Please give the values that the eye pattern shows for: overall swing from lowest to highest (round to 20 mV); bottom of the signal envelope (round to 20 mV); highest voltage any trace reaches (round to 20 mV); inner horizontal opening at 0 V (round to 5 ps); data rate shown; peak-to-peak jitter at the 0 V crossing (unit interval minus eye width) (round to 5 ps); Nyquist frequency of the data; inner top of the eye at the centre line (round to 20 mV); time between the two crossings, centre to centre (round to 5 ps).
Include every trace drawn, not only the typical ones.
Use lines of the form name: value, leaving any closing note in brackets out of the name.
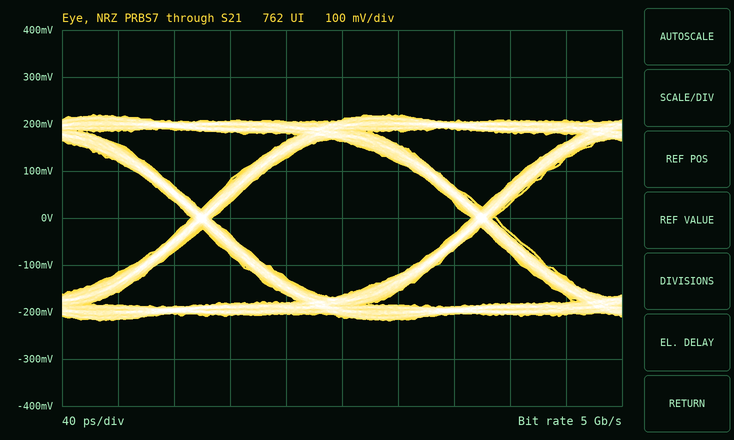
overall swing from lowest to highest: 440 mV
bottom of the signal envelope: -220 mV
highest voltage any trace reaches: 220 mV
inner horizontal opening at 0 V: 185 ps
data rate shown: 5 Gb/s
peak-to-peak jitter at the 0 V crossing (unit interval minus eye width): 15 ps
Nyquist frequency of the data: 2.5 GHz
inner top of the eye at the centre line: 160 mV
time between the two crossings, centre to centre: 200 ps
